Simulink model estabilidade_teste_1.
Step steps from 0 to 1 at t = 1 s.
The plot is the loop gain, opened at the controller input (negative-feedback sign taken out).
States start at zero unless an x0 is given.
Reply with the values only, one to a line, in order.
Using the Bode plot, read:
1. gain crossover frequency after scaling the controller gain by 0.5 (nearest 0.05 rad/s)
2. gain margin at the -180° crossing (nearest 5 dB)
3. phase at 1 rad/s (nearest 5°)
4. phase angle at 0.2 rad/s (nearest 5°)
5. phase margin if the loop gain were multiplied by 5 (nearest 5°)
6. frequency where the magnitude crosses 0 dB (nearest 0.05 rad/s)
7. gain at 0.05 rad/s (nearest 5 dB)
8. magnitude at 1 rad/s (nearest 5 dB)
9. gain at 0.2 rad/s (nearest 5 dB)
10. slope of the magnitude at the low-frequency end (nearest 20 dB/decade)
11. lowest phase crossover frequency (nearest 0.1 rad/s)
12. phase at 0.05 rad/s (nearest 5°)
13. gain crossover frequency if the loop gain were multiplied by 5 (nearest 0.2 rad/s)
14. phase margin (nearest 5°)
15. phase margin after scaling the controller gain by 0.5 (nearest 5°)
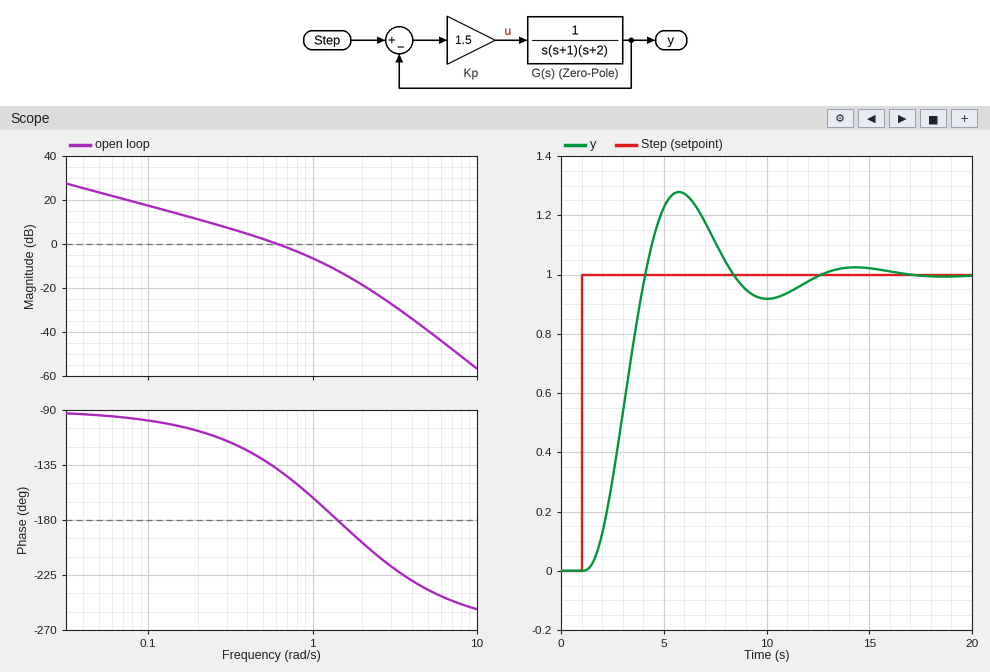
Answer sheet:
0.35 rad/s
10 dB
-160°
-105°
-5°
0.60 rad/s
25 dB
-5 dB
10 dB
-20 dB/decade
1.4 rad/s
-95°
1.6 rad/s
40°
60°
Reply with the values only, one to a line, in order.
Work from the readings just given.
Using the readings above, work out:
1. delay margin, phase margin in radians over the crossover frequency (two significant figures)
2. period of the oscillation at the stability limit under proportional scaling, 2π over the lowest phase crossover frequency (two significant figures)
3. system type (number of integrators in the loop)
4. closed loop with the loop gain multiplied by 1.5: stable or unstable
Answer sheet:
1.2 s
4.5 s
1
stable
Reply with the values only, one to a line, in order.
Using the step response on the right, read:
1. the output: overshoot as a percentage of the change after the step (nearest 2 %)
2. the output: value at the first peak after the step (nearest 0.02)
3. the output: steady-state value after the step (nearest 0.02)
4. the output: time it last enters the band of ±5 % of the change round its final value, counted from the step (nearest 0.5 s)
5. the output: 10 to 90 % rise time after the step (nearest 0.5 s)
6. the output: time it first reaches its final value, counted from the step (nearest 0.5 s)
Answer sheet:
28 %
1.28
1.00
10.5 s
2.0 s
3.0 s
